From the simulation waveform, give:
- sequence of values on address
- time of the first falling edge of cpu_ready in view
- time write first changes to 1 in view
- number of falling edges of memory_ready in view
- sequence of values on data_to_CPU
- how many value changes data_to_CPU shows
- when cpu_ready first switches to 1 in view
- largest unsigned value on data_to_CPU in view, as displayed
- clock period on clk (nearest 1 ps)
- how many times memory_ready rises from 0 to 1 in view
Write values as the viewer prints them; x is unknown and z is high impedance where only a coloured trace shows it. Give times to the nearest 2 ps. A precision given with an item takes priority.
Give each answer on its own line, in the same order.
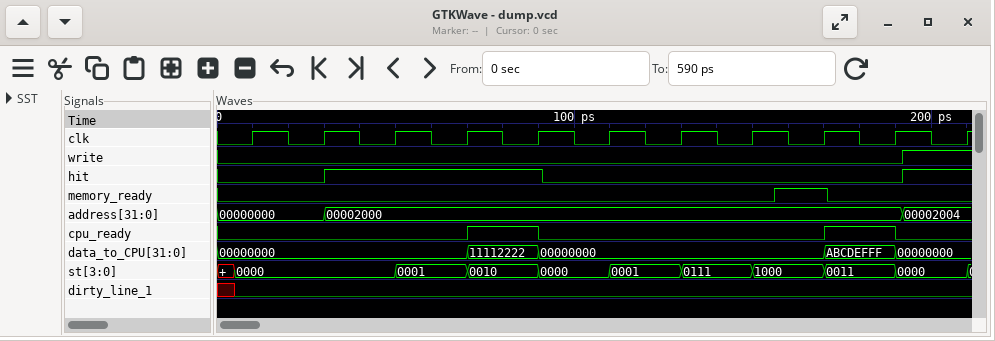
00000000, 00002000, 00002004
90 ps
192 ps
1
00000000, 11112222, 00000000, ABCDEFFF, 00000000
4
70 ps
ABCDEFFF
20 ps
1
